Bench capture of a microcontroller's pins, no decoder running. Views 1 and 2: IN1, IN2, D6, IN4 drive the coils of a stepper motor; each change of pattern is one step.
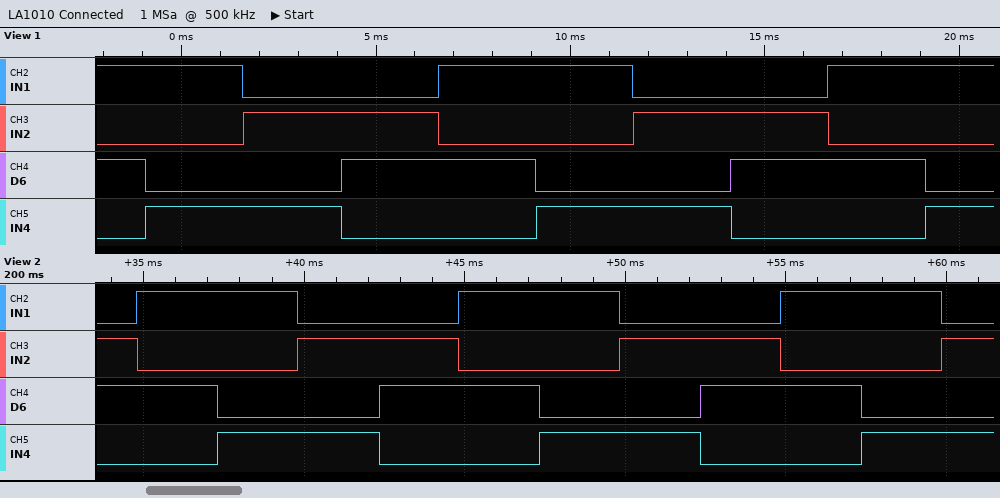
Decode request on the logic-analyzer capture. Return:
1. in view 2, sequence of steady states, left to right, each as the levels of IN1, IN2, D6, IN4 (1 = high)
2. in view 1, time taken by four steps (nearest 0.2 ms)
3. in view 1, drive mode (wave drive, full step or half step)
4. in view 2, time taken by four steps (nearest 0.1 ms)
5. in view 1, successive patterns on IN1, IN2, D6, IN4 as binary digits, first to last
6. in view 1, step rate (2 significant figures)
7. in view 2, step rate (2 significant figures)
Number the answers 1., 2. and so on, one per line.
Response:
1. 0110 1010 1001 0101 0110 1010 1001 0101 0110 1010 1001 0101
2. 10.0 ms
3. full step
4. 10.0 ms
5. 1010 1001 0101 0110 1010 1001 0101 0110 1010 1001
6. 400 steps/s
7. 400 steps/s
